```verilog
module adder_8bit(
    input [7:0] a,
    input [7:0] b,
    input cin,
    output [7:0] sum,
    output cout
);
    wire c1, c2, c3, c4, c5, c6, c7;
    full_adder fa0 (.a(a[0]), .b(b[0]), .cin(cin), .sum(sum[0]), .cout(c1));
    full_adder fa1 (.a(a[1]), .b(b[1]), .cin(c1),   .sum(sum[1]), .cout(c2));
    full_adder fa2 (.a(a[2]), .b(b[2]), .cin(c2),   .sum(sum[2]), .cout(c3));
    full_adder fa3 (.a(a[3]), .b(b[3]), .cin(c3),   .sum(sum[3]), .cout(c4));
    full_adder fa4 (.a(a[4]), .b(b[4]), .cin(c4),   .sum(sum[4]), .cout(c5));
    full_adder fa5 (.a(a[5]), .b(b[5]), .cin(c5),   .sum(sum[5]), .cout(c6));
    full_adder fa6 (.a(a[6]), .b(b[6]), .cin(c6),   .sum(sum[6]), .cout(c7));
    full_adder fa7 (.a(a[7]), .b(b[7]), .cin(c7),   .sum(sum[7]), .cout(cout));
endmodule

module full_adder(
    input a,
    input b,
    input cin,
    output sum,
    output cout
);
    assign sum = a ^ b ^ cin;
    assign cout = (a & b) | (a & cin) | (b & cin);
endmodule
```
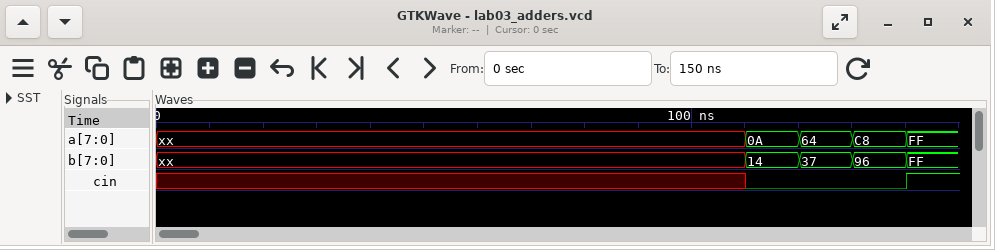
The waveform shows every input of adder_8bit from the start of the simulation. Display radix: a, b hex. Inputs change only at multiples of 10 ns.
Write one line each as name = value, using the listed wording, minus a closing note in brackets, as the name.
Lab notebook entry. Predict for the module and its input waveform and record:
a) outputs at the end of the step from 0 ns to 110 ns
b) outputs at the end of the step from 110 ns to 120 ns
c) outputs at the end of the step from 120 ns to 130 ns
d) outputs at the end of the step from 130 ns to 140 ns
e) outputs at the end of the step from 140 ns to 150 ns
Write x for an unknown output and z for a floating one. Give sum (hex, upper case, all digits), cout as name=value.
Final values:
outputs at the end of the step from 0 ns to 110 ns = sum=x, cout=x
outputs at the end of the step from 110 ns to 120 ns = sum=1E, cout=0
outputs at the end of the step from 120 ns to 130 ns = sum=9B, cout=0
outputs at the end of the step from 130 ns to 140 ns = sum=5E, cout=1
outputs at the end of the step from 140 ns to 150 ns = sum=FF, cout=1
